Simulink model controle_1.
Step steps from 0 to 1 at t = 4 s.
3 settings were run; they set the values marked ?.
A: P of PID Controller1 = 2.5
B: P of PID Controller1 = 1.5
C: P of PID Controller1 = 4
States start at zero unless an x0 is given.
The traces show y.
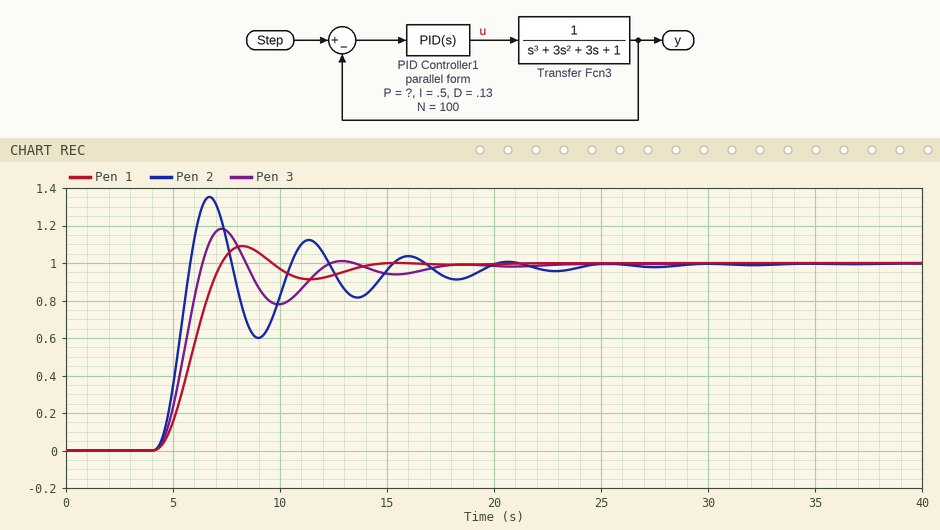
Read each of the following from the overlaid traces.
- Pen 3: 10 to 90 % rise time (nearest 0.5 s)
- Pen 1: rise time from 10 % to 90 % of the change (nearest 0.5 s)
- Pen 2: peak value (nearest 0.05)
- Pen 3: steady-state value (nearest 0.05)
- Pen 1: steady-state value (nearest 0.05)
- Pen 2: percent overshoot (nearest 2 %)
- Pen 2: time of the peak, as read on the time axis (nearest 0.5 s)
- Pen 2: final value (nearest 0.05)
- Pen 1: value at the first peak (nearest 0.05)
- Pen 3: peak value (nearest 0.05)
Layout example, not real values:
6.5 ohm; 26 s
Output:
1.5 s; 2.0 s; 1.35; 1.00; 1.00; 36 %; 6.5 s; 1.00; 1.10; 1.20
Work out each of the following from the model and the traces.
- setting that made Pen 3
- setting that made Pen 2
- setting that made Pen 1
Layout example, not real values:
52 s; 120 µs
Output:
A; C; B
